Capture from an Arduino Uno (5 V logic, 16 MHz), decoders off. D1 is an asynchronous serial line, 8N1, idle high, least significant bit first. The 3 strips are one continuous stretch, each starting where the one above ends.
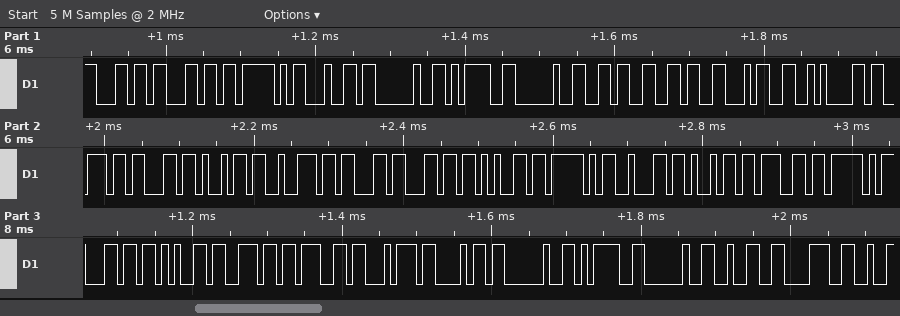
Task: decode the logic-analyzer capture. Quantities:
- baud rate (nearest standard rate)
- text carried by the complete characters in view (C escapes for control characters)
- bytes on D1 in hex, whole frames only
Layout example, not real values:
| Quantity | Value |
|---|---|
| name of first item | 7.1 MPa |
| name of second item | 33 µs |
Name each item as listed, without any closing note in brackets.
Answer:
| Quantity | Value |
|---|---|
| baud rate | 115200 baud |
| text carried by the complete characters in view | "ll_d = 664\nscircle_big_length = 28" |
| bytes on D1 in hex, whole frames only | 6C 6C 5F 64 20 3D 20 36 36 34 0A 73 63 69 72 63 6C 65 5F 62 69 67 5F 6C 65 6E 67 74 68 20 3D 20 32 38 |
